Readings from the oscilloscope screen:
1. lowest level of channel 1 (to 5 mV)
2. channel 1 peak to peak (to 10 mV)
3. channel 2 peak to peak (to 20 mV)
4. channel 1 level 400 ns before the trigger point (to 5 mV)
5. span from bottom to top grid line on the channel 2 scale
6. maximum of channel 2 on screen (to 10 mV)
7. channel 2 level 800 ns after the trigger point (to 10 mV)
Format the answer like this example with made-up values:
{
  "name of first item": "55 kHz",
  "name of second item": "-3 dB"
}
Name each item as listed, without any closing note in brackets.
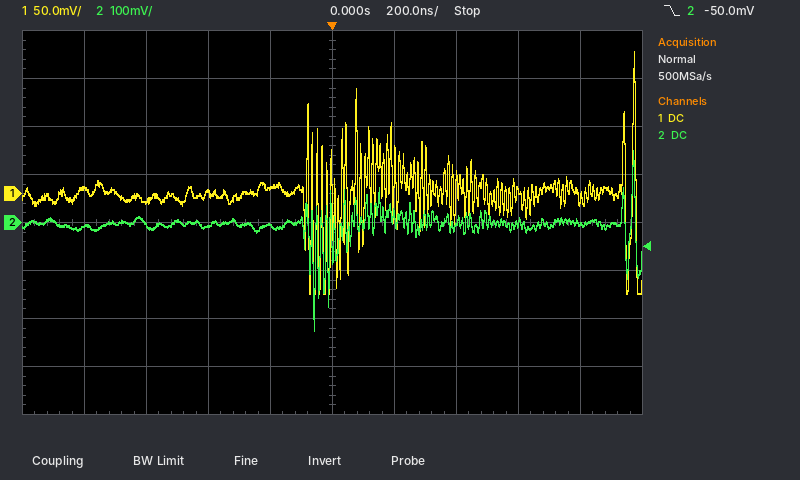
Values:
{
  "lowest level of channel 1": "-105 mV",
  "channel 1 peak to peak": "250 mV",
  "channel 2 peak to peak": "380 mV",
  "channel 1 level 400 ns before the trigger point": "0 mV",
  "span from bottom to top grid line on the channel 2 scale": "800 mV",
  "maximum of channel 2 on screen": "150 mV",
  "channel 2 level 800 ns after the trigger point": "0 mV"
}
